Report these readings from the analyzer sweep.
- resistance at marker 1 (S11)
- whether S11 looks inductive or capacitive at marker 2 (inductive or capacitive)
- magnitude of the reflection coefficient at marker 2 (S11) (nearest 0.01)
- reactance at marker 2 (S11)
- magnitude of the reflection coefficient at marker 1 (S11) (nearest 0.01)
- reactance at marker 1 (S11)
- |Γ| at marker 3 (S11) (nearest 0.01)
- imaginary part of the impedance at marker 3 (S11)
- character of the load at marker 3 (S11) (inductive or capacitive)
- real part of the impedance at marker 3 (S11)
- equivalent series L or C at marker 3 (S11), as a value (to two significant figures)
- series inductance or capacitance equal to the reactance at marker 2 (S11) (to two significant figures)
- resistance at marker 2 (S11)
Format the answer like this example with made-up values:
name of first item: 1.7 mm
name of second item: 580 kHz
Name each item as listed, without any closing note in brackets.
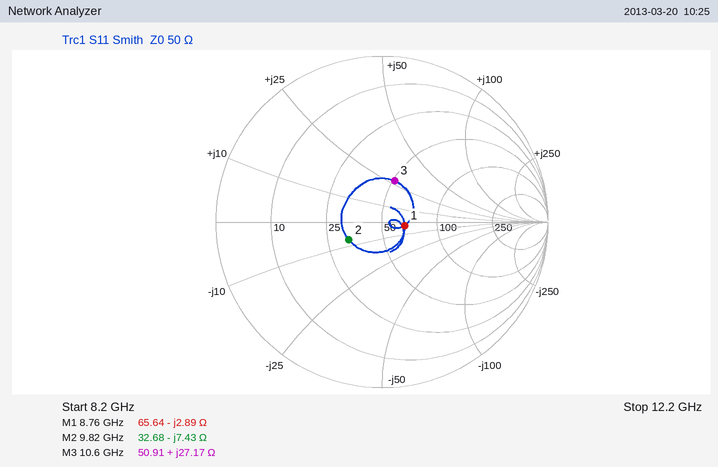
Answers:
resistance at marker 1: 65.64 Ω
whether S11 looks inductive or capacitive at marker 2: capacitive
magnitude of the reflection coefficient at marker 2 (S11): 0.23
reactance at marker 2: -7.43 Ω
magnitude of the reflection coefficient at marker 1 (S11): 0.14
reactance at marker 1: -2.89 Ω
|Γ| at marker 3 (S11): 0.26
imaginary part of the impedance at marker 3: +27.17 Ω
character of the load at marker 3 (S11): inductive
real part of the impedance at marker 3: 50.91 Ω
equivalent series L or C at marker 3 (S11), as a value: 410 pH
series inductance or capacitance equal to the reactance at marker 2 (S11): 2.2 pF
resistance at marker 2: 32.68 Ω
